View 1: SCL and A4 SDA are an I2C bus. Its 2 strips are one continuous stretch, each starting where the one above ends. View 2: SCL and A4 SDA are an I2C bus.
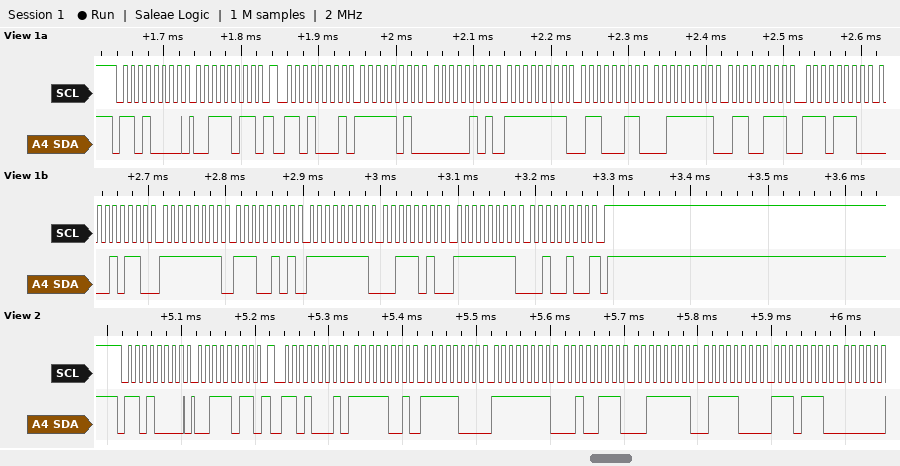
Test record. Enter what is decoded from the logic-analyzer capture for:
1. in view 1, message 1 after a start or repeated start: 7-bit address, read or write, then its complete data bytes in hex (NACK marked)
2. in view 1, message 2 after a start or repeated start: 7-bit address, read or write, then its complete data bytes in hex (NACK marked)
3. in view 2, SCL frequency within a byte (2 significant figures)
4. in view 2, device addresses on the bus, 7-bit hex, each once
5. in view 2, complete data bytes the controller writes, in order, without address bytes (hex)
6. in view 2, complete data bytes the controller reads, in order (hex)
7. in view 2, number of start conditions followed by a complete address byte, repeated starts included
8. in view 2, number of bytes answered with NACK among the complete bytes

0x68 write: 3B
0x68 read: FA 05 FF 63 3F 67 EE 16 FF E5 FF 3A FF 24 NACK
100 kHz
0x68
3B
F9 F8 FF 27 3F 78 EE
2
0
